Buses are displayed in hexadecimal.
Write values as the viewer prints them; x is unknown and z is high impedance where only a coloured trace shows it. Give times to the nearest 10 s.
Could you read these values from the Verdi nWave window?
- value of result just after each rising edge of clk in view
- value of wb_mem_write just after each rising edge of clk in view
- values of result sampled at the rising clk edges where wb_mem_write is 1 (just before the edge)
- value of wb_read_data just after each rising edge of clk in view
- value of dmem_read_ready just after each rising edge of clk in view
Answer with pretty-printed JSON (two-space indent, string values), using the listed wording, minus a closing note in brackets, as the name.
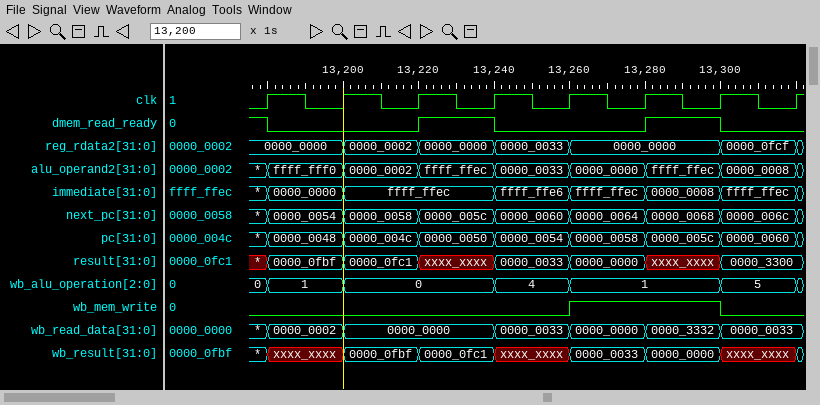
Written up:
{
  "value of result just after each rising edge of clk in view": "0000_0fbf, 0000_0fc1, xxxx_xxxx, 0000_0033, 0000_0000, xxxx_xxxx, 0000_3300, 0000_3300",
  "value of wb_mem_write just after each rising edge of clk in view": "0 0 0 0 1 1 0 0",
  "values of result sampled at the rising clk edges where wb_mem_write is 1": "0000_0000, xxxx_xxxx",
  "value of wb_read_data just after each rising edge of clk in view": "0000_0002, 0000_0000, 0000_0000, 0000_0033, 0000_0000, 0000_3332, 0000_0033, 0000_0033",
  "value of dmem_read_ready just after each rising edge of clk in view": "0 0 1 0 0 1 0 0"
}
